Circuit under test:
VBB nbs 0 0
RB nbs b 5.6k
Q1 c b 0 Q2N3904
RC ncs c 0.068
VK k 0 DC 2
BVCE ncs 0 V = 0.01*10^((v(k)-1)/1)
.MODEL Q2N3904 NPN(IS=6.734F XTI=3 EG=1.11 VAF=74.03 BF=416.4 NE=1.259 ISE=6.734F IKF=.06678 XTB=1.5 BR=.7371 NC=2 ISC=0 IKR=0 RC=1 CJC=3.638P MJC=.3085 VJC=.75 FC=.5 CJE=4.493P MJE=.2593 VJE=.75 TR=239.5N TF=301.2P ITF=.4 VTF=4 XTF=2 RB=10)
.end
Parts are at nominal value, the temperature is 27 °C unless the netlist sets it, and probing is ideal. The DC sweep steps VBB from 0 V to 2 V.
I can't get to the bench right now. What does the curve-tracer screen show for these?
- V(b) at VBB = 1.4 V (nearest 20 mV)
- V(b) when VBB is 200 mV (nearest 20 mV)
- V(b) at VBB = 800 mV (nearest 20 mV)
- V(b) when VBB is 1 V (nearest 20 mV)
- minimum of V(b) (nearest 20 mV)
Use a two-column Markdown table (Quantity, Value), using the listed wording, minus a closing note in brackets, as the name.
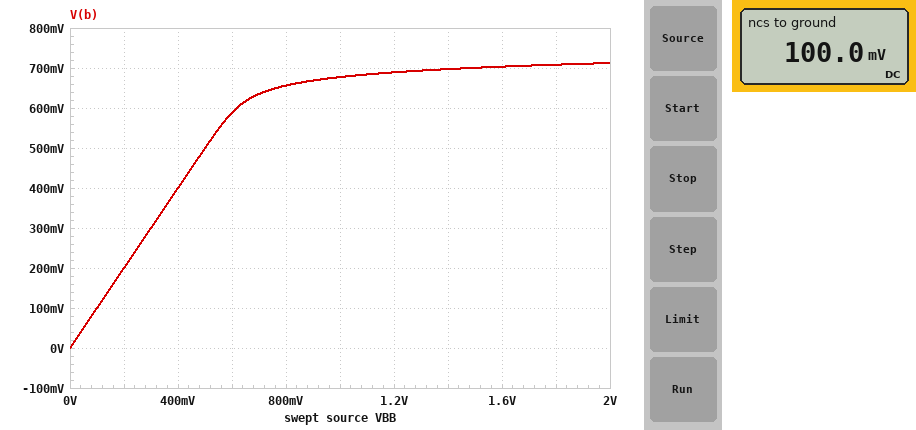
| Quantity | Value |
|---|---|
| V(b) at VBB = 1.4 V | 700 mV |
| V(b) when VBB is 200 mV | 200 mV |
| V(b) at VBB = 800 mV | 660 mV |
| V(b) when VBB is 1 V | 680 mV |
| minimum of V(b) | 0 V |
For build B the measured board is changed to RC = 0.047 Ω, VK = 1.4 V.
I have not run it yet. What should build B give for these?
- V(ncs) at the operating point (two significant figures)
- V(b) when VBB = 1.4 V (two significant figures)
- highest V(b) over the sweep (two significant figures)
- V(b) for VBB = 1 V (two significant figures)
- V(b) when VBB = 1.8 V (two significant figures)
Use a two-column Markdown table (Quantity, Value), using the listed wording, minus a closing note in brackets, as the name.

| Quantity | Value |
|---|---|
| V(ncs) at the operating point | 25 mV |
| V(b) when VBB = 1.4 V | 630 mV |
| highest V(b) over the sweep | 650 mV |
| V(b) for VBB = 1 V | 610 mV |
| V(b) when VBB = 1.8 V | 640 mV |
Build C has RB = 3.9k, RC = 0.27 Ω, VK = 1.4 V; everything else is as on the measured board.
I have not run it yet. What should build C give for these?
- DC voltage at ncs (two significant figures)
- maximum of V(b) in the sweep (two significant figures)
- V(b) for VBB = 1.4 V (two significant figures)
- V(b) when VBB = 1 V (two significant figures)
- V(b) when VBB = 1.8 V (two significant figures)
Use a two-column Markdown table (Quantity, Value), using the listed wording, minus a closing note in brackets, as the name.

| Quantity | Value |
|---|---|
| DC voltage at ncs | 25 mV |
| maximum of V(b) in the sweep | 660 mV |
| V(b) for VBB = 1.4 V | 640 mV |
| V(b) when VBB = 1 V | 620 mV |
| V(b) when VBB = 1.8 V | 650 mV |
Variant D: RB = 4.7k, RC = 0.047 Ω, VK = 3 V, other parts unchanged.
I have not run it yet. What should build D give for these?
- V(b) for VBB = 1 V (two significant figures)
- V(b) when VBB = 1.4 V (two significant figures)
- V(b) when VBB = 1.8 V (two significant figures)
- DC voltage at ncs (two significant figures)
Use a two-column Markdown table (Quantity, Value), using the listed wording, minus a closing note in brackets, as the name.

| Quantity | Value |
|---|---|
| V(b) for VBB = 1 V | 730 mV |
| V(b) when VBB = 1.4 V | 750 mV |
| V(b) when VBB = 1.8 V | 770 mV |
| DC voltage at ncs | 1.0 V |
